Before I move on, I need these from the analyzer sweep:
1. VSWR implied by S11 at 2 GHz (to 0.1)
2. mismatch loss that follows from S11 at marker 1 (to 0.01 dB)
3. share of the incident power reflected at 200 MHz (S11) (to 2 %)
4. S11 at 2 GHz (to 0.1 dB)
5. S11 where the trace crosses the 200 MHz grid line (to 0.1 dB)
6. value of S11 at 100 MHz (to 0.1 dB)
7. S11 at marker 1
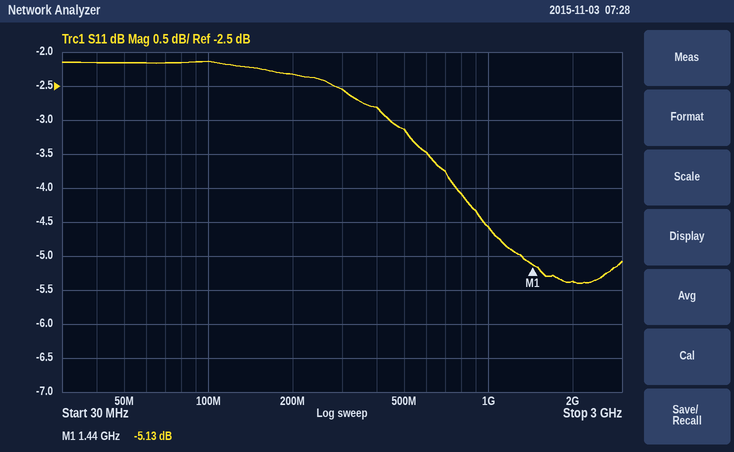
3.3
1.59 dB
58 %
-5.4 dB
-2.3 dB
-2.1 dB
-5.13 dB
